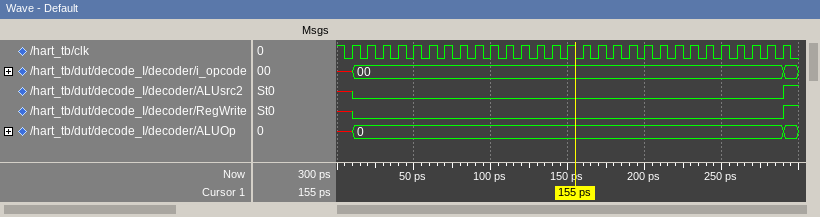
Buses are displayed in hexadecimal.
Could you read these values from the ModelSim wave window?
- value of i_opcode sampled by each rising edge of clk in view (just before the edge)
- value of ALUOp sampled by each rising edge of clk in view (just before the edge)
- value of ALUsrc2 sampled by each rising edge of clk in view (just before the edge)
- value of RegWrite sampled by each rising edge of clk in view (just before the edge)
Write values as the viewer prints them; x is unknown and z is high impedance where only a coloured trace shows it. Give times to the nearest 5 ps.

x, 00, 00, 00, 00, 00, 00, 00, 00, 00, 00, 00, 00, 00, 00, 00, 00, 00, 00, 00, 00, 00, 00, 00, 00, 00, 00, 00, 00
x, 0, 0, 0, 0, 0, 0, 0, 0, 0, 0, 0, 0, 0, 0, 0, 0, 0, 0, 0, 0, 0, 0, 0, 0, 0, 0, 0, 0
x 0 0 0 0 0 0 0 0 0 0 0 0 0 0 0 0 0 0 0 0 0 0 0 0 0 0 0 0
x 0 0 0 0 0 0 0 0 0 0 0 0 0 0 0 0 0 0 0 0 0 0 0 0 0 0 0 0
